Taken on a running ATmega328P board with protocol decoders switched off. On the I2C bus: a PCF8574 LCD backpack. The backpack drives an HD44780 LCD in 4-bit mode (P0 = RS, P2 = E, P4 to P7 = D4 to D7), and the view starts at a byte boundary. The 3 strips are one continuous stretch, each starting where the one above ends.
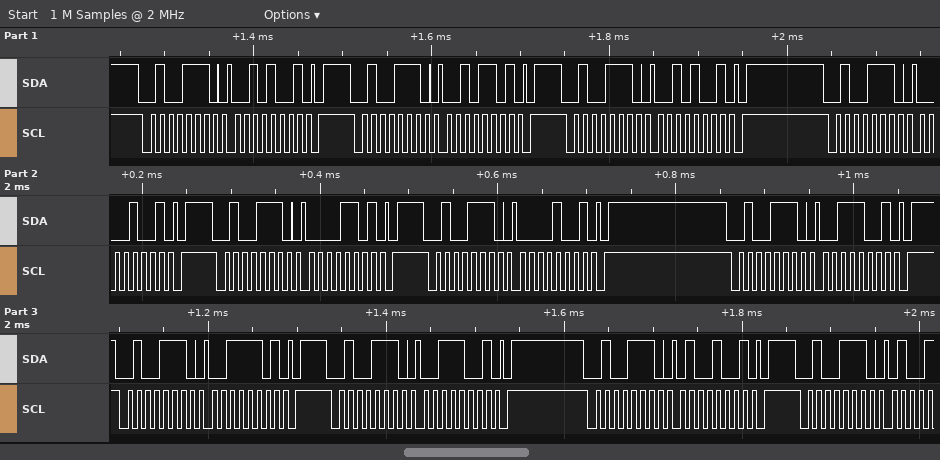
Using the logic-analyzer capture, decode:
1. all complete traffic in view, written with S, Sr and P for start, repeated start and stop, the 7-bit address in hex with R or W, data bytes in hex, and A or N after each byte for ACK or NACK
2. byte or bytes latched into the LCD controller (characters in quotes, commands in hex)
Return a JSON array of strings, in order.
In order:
["S 27W A 29 A P S 27W A 2D A P S 27W A 29 A P S 27W A 09 A P S 27W A 0D A P S 27W A 09 A P S 27W A 39 A P S 27W A 3D A P S 27W A 39 A P S 27W A 49 A P S 27W A", "' '"]
